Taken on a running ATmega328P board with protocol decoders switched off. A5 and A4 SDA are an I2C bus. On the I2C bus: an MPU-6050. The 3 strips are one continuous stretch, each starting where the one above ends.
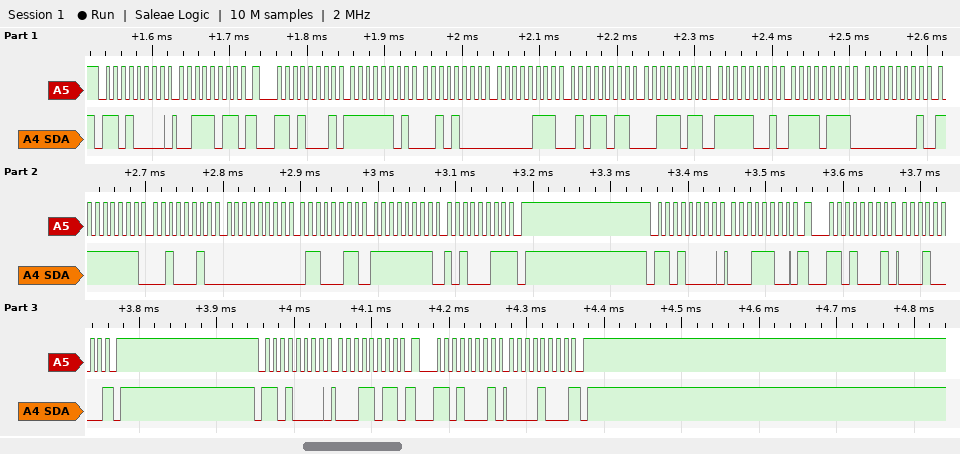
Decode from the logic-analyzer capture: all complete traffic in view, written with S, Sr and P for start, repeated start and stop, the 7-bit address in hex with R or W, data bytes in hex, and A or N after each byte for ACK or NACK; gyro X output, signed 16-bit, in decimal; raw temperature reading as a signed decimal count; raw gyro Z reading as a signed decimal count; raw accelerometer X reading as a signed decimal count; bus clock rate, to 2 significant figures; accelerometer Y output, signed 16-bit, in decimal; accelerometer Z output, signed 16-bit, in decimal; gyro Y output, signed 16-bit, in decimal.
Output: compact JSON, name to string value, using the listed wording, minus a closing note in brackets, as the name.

{"all complete traffic in view, written with S, Sr and P for start, repeated start and stop, the 7-bit address in hex with R or W, data bytes in hex, and A or N after each byte for ACK or NACK": "S 68W A 3B A Sr 68R A FD A 28 A 07 A 5B A 3B A F9 A F7 A 01 A FF A 22 A 00 A 63 A FF A A3 N P S 68W A 1C A Sr 68R A 10 N P S 68W A 1B A Sr 68R A 08 N P", "gyro X output, signed 16-bit, in decimal": "-222", "raw temperature reading as a signed decimal count": "-2303", "raw gyro Z reading as a signed decimal count": "-93", "raw accelerometer X reading as a signed decimal count": "-728", "bus clock rate, to 2 significant figures": "100 kHz", "accelerometer Y output, signed 16-bit, in decimal": "1883", "accelerometer Z output, signed 16-bit, in decimal": "15353", "gyro Y output, signed 16-bit, in decimal": "99"}
